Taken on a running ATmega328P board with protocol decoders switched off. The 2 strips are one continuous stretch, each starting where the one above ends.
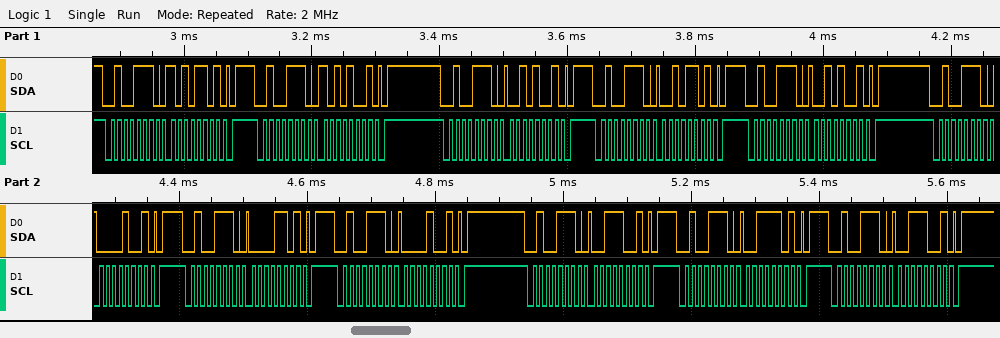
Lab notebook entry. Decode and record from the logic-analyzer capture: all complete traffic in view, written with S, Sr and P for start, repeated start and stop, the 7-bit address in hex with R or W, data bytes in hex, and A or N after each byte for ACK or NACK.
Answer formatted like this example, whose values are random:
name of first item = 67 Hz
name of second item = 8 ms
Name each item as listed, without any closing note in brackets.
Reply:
all complete traffic in view, written with S, Sr and P for start, repeated start and stop, the 7-bit address in hex with R or W, data bytes in hex, and A or N after each byte for ACK or NACK = S 27W A AD A P S 27W A A9 A P S 27W A 29 A P S 27W A 2D A P S 27W A 29 A P S 27W A 09 A P S 27W A 0D A P S 27W A 09 A P S 27W A 39 A P S 27W A 3D A P S 27W A 39 A P
